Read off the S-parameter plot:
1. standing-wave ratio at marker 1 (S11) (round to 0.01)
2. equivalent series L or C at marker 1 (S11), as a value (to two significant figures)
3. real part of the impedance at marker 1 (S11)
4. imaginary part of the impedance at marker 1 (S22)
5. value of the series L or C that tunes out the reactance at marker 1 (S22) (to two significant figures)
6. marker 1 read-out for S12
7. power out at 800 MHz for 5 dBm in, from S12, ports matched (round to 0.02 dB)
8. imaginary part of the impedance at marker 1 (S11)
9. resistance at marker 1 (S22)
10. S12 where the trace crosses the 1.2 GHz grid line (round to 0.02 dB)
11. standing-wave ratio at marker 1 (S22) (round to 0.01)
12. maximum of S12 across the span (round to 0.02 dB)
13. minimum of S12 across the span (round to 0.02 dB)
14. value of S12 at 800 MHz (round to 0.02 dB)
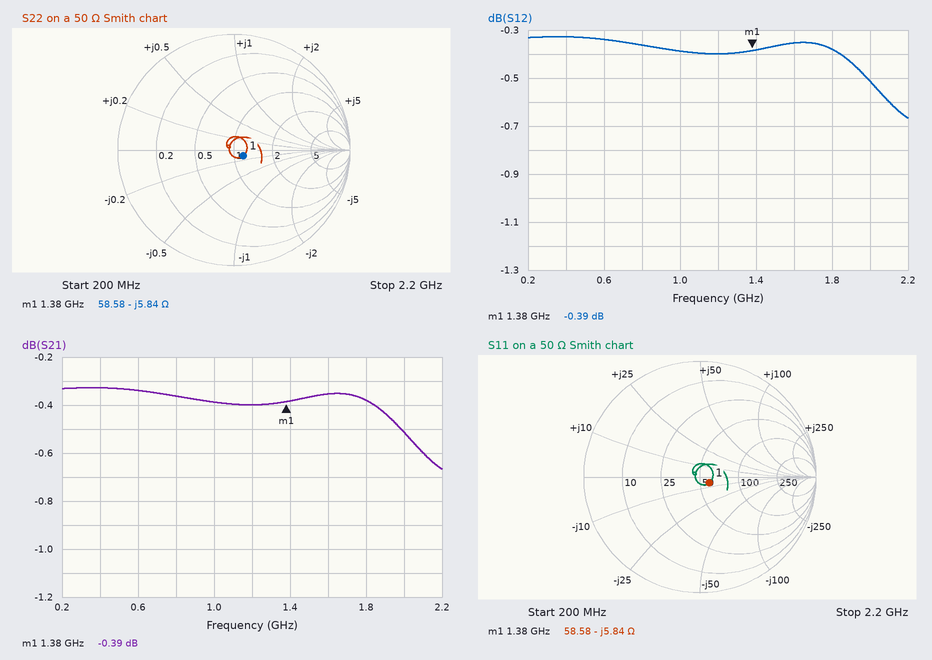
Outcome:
1.21
20 pF
58.58 Ω
-5.84 Ω
670 pH
-0.39 dB
4.64 dBm
-5.84 Ω
58.58 Ω
-0.40 dB
1.21
-0.32 dB
-0.66 dB
-0.36 dB
